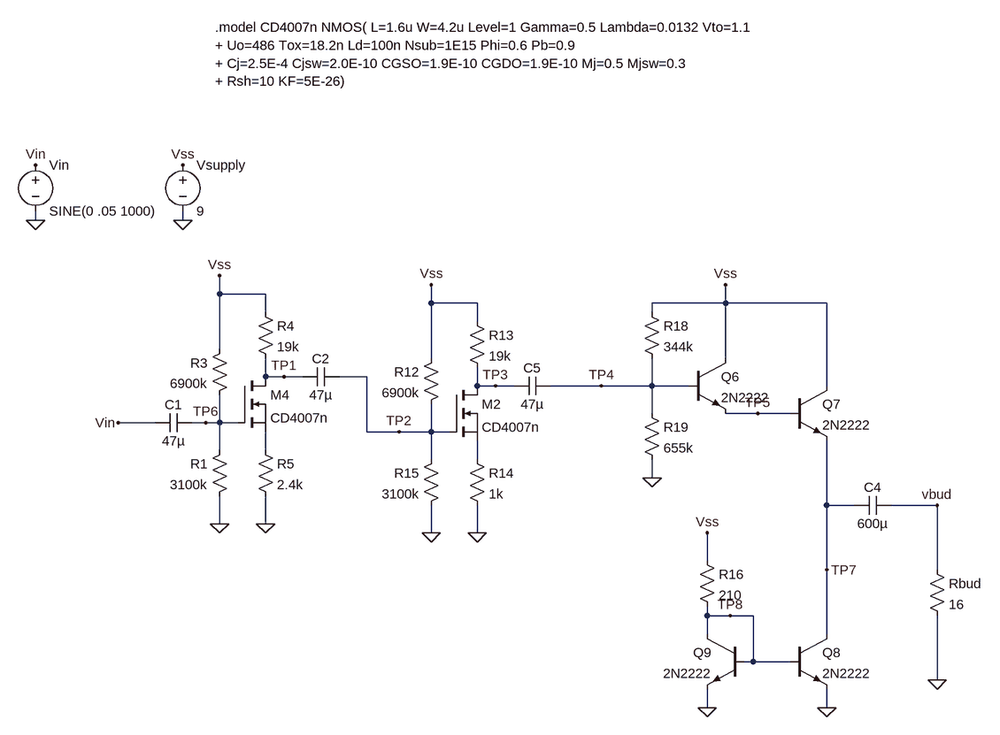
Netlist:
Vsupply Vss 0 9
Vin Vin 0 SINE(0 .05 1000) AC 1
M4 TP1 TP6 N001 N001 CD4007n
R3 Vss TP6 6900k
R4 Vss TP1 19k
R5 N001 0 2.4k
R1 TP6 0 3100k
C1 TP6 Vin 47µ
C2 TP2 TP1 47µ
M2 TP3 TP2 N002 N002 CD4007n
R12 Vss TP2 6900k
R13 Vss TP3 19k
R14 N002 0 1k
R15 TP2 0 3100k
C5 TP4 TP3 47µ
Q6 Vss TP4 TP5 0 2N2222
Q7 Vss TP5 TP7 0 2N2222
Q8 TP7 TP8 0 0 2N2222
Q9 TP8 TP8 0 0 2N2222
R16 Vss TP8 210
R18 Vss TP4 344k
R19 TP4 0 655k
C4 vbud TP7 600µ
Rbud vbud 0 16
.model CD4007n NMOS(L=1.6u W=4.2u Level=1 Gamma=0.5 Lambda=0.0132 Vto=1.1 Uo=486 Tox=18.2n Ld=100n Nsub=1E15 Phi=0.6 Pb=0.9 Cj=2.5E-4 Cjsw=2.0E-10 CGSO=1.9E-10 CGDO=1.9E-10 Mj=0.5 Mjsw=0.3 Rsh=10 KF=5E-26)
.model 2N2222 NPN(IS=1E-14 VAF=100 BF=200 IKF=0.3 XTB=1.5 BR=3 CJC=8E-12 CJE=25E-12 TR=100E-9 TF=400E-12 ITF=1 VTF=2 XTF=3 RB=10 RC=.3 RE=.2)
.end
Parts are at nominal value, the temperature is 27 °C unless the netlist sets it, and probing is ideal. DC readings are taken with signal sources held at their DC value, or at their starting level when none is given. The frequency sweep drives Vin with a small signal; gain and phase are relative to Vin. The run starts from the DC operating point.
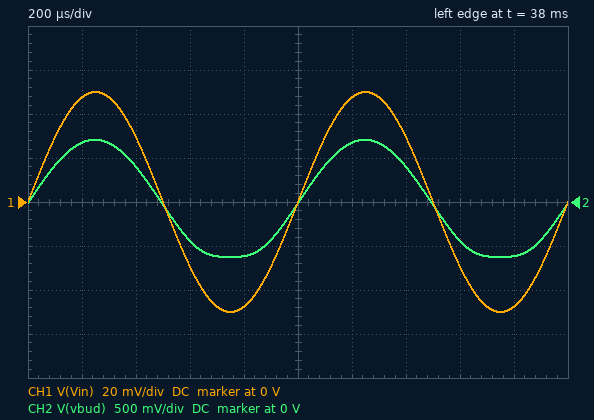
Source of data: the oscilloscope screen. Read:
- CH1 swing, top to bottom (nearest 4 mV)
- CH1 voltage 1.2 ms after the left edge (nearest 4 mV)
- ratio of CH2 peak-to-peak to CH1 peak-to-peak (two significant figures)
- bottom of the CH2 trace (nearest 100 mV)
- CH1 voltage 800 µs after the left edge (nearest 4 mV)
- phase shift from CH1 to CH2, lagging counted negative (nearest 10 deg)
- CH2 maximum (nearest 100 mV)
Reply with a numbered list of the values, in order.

1. 100 mV
2. 48 mV
3. 13
4. -600 mV
5. -48 mV
6. 0 deg
7. 700 mV
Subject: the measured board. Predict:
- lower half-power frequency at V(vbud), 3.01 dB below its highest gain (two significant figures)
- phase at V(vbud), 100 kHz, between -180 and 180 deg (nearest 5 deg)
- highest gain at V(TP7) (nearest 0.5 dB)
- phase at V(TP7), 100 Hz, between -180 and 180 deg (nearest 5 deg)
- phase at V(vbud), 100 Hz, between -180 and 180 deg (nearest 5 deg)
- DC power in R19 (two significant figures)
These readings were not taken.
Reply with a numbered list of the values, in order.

1. 15 Hz
2. -5 deg
3. 24.5 dB
4. 0 deg
5. 10 deg
6. 49 µW
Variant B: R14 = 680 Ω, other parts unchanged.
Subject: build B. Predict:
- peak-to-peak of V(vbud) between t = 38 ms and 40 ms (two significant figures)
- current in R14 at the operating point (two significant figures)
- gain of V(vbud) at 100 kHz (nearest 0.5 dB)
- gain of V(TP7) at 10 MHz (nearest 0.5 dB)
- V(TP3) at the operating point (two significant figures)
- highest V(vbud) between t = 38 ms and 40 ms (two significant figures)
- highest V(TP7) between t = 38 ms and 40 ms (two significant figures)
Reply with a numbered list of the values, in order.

1. 1.4 V
2. 310 µA
3. 24.5 dB
4. 2.5 dB
5. 3.1 V
6. 780 mV
7. 5.1 V
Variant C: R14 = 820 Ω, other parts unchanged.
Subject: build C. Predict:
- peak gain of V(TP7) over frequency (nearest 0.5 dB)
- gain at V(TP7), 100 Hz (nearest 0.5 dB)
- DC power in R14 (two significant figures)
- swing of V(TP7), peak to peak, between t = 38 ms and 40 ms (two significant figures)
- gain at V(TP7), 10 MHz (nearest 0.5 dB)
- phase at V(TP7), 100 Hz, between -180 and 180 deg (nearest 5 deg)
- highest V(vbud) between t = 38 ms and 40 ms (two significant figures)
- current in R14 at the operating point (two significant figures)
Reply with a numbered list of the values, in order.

1. 25.0 dB
2. 24.0 dB
3. 73 µW
4. 1.4 V
5. 2.0 dB
6. 0 deg
7. 750 mV
8. 300 µA
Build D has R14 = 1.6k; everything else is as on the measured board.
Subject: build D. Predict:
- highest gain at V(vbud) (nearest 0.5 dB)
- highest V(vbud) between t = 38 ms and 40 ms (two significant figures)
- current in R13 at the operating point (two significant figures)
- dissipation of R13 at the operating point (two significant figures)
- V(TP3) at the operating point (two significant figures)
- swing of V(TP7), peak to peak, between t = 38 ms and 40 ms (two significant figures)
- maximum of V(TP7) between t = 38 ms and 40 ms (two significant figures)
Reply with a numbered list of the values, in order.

1. 21.5 dB
2. 590 mV
3. 240 µA
4. 1.1 mW
5. 4.4 V
6. 1.2 V
7. 4.9 V
